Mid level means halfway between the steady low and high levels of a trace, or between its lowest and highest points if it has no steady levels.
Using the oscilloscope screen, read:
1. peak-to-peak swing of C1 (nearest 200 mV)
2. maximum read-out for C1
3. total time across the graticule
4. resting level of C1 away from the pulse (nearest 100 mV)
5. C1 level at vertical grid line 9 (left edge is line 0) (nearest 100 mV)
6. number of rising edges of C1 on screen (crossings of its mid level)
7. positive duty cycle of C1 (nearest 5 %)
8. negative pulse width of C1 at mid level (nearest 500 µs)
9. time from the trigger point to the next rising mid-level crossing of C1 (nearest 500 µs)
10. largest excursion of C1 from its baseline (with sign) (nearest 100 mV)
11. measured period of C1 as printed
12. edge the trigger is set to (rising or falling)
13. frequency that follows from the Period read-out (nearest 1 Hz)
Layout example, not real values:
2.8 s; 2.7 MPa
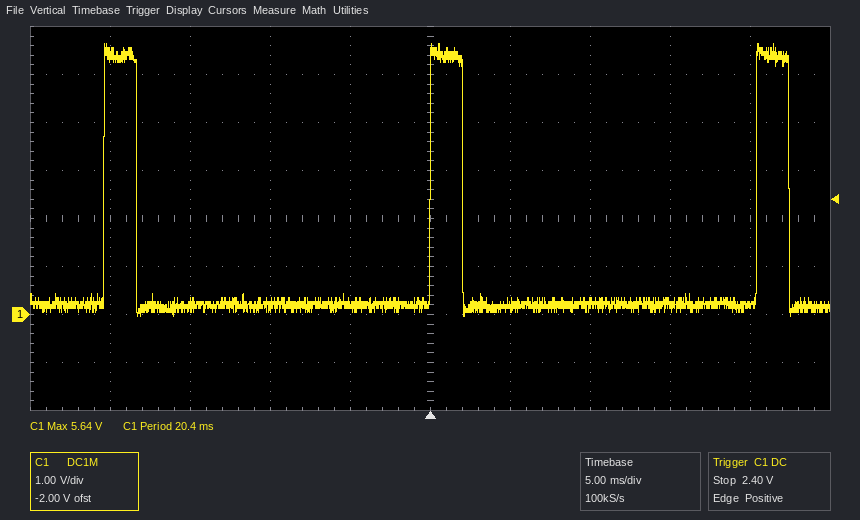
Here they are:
5.6 V; 5.64 V; 50 ms; 200 mV; 200 mV; 3; 10 %; 18.5 ms; 20.5 ms; +5.4 V; 20.4 ms; rising; 49 Hz
